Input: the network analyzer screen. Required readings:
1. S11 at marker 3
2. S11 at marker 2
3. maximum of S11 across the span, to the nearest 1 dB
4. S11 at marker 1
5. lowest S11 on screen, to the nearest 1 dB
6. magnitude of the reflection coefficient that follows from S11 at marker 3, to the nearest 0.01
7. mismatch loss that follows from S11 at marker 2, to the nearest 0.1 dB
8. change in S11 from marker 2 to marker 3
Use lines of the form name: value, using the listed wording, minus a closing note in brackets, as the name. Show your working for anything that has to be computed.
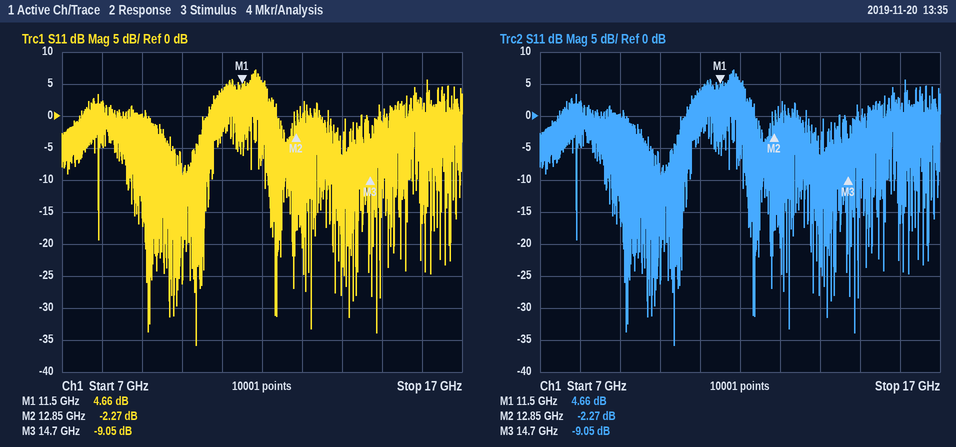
S11 at marker 3: -9.05 dB
S11 at marker 2: -2.27 dB
maximum of S11 across the span, to the nearest 1 dB: 7 dB
S11 at marker 1: 4.66 dB
lowest S11 on screen, to the nearest 1 dB: -36 dB
magnitude of the reflection coefficient that follows from S11 at marker 3, to the nearest 0.01: 10^(-9.05/20) ≈ 0.35
mismatch loss that follows from S11 at marker 2, to the nearest 0.1 dB: −10 log10(1 − 10^(-2.27/10)) ≈ 3.9 dB
change in S11 from marker 2 to marker 3: -9.05 − (-2.27) = -6.78 dB
